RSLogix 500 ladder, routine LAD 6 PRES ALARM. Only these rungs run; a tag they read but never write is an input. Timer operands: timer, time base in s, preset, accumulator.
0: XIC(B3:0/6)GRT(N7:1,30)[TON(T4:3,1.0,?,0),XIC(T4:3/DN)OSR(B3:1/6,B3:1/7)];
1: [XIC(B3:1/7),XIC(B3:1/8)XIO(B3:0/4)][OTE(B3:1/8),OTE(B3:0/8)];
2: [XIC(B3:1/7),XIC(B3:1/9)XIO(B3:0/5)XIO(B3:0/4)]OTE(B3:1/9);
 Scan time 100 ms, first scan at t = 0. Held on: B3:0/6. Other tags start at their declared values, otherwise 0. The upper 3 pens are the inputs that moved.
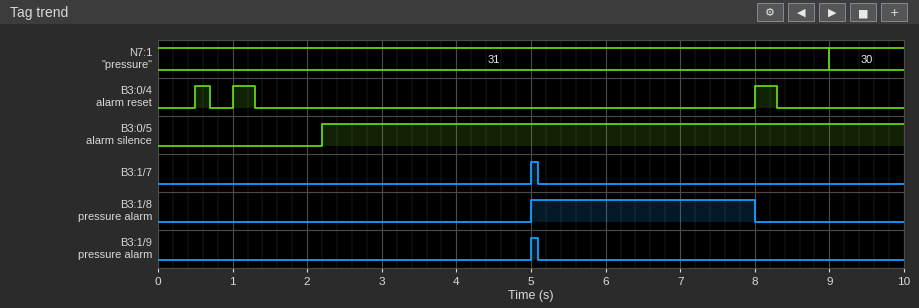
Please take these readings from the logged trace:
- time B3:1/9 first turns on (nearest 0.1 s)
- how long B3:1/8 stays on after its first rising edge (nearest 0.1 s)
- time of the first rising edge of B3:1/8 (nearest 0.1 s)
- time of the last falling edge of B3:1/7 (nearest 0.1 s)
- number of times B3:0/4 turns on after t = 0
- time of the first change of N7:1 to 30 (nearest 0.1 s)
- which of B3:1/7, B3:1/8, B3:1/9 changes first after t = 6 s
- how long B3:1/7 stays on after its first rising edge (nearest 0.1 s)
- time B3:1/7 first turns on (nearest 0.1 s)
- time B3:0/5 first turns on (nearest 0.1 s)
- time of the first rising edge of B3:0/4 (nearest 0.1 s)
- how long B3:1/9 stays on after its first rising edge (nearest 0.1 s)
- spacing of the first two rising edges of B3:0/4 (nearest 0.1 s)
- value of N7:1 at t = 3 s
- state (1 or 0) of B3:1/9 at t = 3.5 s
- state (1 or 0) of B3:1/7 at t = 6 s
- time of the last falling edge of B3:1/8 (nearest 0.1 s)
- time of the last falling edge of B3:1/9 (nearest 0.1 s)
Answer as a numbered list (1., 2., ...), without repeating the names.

1. 5.0 s
2. 3.0 s
3. 5.0 s
4. 5.1 s
5. 3
6. 9.0 s
7. B3:1/8
8. 0.1 s
9. 5.0 s
10. 2.2 s
11. 0.5 s
12. 0.1 s
13. 0.5 s
14. 31
15. 0
16. 0
17. 8.0 s
18. 5.1 s
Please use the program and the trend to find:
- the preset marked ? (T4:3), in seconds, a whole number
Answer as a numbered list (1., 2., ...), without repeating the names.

1. 5 s
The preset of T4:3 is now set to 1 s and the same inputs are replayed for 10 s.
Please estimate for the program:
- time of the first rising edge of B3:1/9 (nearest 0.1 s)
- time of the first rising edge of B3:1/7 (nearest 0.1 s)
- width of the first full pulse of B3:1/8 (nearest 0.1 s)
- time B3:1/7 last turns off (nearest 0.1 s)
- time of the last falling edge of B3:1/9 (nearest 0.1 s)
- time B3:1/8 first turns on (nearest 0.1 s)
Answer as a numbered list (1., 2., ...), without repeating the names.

1. 1.0 s
2. 1.0 s
3. 0.1 s
4. 1.1 s
5. 1.1 s
6. 1.0 s
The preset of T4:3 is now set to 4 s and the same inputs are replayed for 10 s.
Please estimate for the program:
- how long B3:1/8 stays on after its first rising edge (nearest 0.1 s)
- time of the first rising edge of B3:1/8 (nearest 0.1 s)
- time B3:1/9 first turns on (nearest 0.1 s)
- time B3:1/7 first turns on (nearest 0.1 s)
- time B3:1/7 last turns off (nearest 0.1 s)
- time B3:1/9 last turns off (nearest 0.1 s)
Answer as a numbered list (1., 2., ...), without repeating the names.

1. 4.0 s
2. 4.0 s
3. 4.0 s
4. 4.0 s
5. 4.1 s
6. 4.1 s
